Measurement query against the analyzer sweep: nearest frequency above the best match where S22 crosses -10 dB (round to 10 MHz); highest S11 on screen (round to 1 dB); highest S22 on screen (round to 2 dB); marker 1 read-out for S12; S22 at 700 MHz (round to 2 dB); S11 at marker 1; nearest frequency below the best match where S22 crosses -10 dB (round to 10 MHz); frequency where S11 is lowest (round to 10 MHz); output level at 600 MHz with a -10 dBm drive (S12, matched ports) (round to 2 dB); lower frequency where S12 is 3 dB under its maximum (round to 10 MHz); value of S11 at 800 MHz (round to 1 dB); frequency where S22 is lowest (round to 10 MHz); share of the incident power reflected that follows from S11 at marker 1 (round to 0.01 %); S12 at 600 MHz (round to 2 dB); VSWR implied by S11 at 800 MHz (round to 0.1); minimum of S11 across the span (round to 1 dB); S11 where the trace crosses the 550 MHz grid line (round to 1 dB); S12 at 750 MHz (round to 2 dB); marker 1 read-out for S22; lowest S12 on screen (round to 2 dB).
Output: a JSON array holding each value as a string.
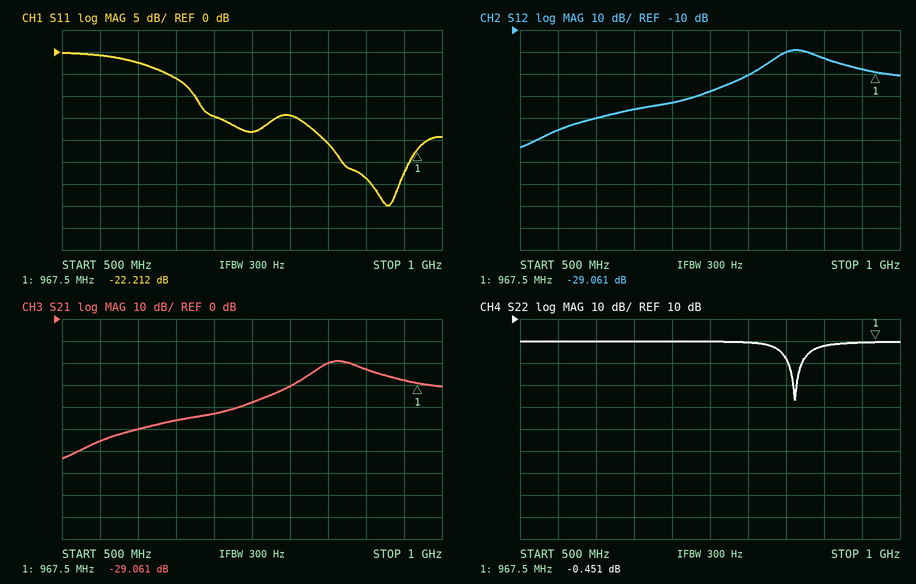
["870 MHz", "0 dB", "0 dB", "-29.061 dB", "0 dB", "-22.212 dB", "850 MHz", "930 MHz", "-60 dBm", "840 MHz", "-14 dB", "860 MHz", "0.60 %", "-50 dB", "1.5", "-35 dB", "-1 dB", "-38 dB", "-0.451 dB", "-64 dB"]
